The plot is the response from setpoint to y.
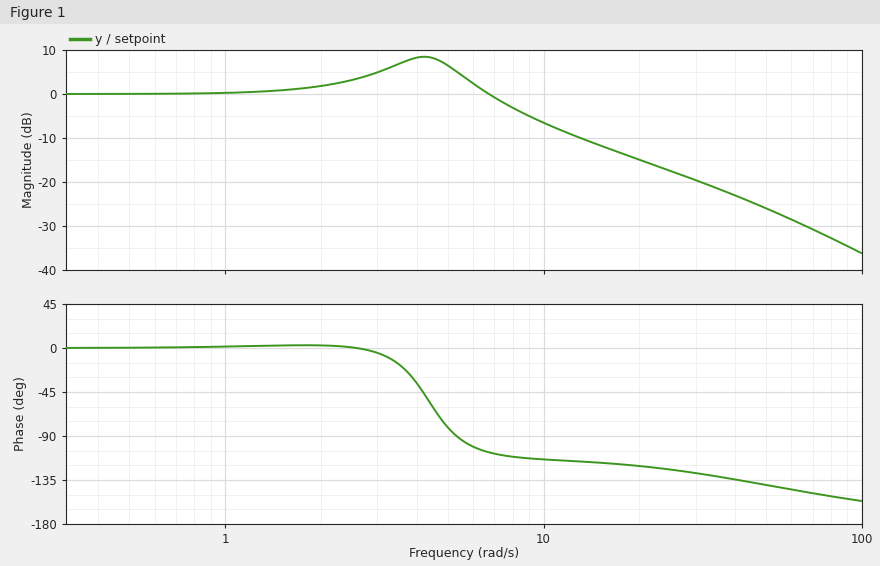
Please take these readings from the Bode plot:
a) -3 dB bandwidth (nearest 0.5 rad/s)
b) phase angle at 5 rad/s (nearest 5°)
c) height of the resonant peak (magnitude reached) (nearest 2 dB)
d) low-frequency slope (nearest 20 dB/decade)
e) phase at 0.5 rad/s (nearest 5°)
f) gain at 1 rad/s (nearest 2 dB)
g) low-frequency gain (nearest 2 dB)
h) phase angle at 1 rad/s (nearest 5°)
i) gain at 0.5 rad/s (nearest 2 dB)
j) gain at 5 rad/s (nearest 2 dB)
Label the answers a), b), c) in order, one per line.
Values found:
a) 8.0 rad/s
b) -80°
c) 8 dB
d) 0 dB/decade
e) 0°
f) 0 dB
g) 0 dB
h) 0°
i) 0 dB
j) 6 dB
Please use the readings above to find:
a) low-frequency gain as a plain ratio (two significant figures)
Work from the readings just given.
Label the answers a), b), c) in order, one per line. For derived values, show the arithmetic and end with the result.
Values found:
a) 10^(0 / 20) = 1.0
